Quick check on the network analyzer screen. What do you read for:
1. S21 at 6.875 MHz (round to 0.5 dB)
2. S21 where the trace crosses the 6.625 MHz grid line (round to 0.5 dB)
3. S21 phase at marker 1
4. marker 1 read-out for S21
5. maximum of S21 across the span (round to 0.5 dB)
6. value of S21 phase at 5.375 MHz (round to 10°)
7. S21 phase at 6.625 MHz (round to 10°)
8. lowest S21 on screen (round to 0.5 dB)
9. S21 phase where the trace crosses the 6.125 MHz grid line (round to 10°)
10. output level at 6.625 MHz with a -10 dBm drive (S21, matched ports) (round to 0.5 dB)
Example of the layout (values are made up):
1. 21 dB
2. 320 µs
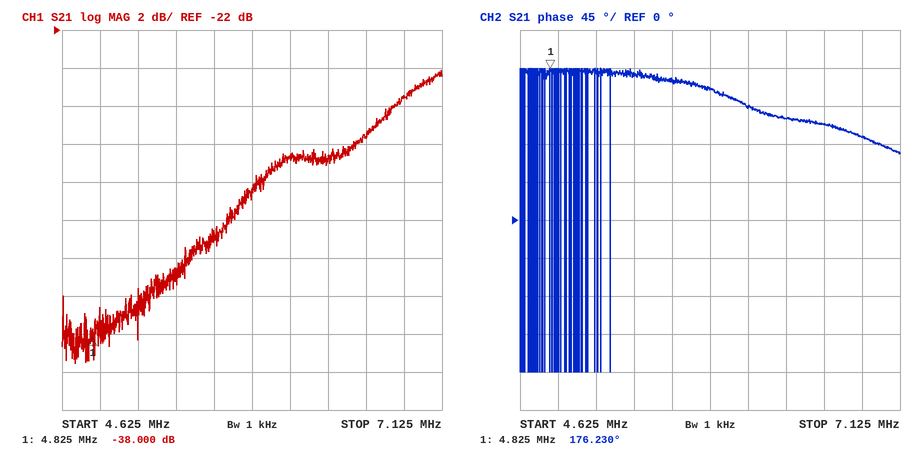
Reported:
1. -25.5 dB
2. -27.5 dB
3. 176.230°
4. -38.000 dB
5. -24.0 dB
6. 170°
7. 110°
8. -39.5 dB
9. 130°
10. -37.5 dBm
